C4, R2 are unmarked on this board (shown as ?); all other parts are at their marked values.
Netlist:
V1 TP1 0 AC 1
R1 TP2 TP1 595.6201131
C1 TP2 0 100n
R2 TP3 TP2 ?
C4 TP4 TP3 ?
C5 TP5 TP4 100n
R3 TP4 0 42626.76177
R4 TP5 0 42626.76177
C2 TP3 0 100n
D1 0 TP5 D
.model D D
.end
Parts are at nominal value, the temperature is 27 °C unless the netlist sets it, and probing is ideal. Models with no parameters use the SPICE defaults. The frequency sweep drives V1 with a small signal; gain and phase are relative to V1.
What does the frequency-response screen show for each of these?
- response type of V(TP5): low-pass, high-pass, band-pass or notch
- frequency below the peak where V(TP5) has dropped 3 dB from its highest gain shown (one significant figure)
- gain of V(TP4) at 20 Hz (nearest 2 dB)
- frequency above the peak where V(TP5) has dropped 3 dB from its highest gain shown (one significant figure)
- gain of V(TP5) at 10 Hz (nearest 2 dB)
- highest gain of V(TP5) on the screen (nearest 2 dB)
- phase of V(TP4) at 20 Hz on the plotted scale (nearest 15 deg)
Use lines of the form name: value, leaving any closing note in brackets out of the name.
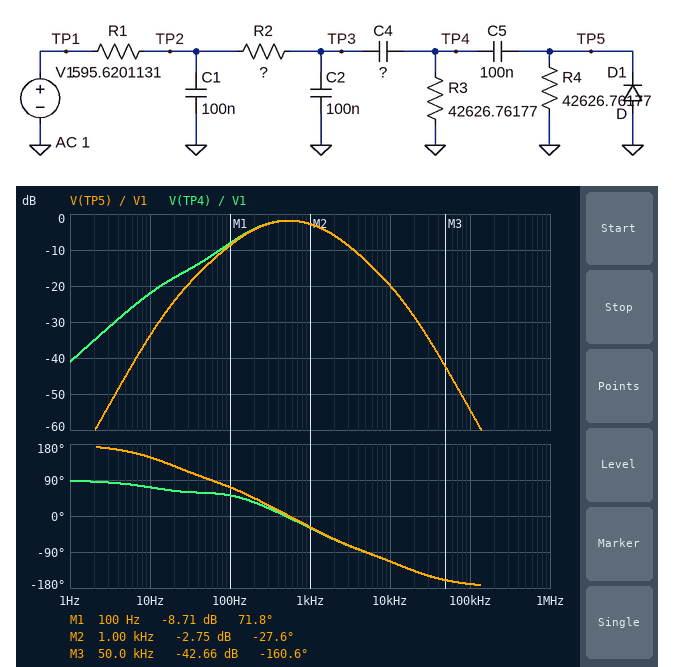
response type of V(TP5): low-pass, high-pass, band-pass or notch: band-pass
frequency below the peak where V(TP5) has dropped 3 dB from its highest gain shown: 200 Hz
gain of V(TP4) at 20 Hz: -18 dB
frequency above the peak where V(TP5) has dropped 3 dB from its highest gain shown: 2 kHz
gain of V(TP5) at 10 Hz: -34 dB
highest gain of V(TP5) on the screen: -2 dB
phase of V(TP4) at 20 Hz on the plotted scale: 60 deg
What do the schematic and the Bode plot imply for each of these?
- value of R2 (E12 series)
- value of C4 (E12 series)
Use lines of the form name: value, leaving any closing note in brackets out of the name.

value of R2: 220 Ω
value of C4: 33 nF
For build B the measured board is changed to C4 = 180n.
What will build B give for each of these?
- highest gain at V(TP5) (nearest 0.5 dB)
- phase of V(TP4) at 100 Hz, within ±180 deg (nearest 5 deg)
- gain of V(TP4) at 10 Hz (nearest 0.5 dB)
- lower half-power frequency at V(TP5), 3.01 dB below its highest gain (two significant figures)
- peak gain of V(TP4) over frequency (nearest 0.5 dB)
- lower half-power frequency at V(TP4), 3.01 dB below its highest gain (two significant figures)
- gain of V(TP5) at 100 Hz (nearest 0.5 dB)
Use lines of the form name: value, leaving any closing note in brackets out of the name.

highest gain at V(TP5): -1.0 dB
phase of V(TP4) at 100 Hz, within ±180 deg: 15 deg
gain of V(TP4) at 10 Hz: -8.5 dB
lower half-power frequency at V(TP5), 3.01 dB below its highest gain: 61 Hz
peak gain of V(TP4) over frequency: -0.5 dB
lower half-power frequency at V(TP4), 3.01 dB below its highest gain: 38 Hz
gain of V(TP5) at 100 Hz: -2.0 dB
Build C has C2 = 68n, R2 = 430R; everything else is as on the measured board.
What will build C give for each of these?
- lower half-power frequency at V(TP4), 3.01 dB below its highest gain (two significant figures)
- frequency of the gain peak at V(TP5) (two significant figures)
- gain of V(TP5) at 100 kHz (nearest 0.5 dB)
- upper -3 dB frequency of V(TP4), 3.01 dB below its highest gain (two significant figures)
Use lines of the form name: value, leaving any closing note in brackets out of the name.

lower half-power frequency at V(TP4), 3.01 dB below its highest gain: 180 Hz
frequency of the gain peak at V(TP5): 580 Hz
gain of V(TP5) at 100 kHz: -57.0 dB
upper -3 dB frequency of V(TP4), 3.01 dB below its highest gain: 1.8 kHz
